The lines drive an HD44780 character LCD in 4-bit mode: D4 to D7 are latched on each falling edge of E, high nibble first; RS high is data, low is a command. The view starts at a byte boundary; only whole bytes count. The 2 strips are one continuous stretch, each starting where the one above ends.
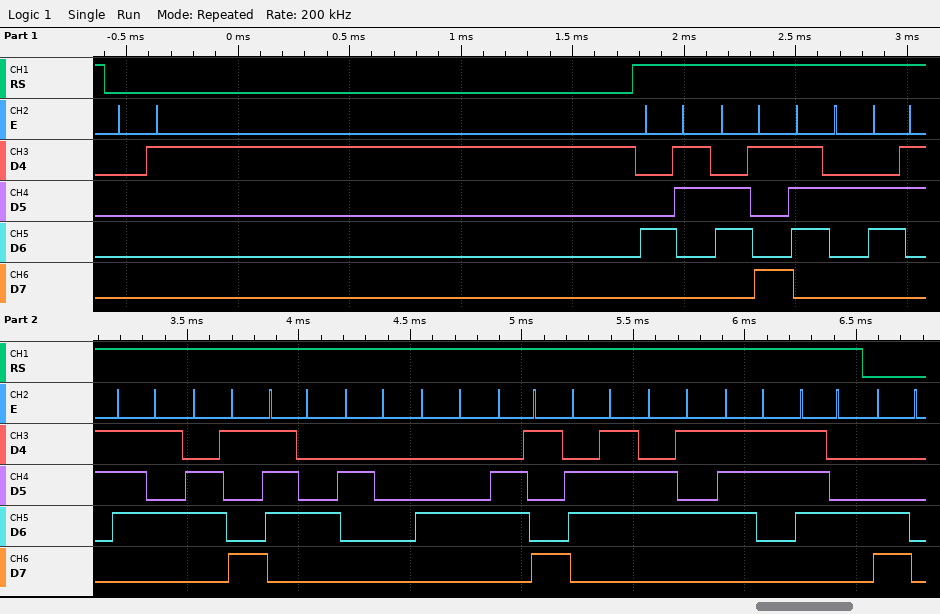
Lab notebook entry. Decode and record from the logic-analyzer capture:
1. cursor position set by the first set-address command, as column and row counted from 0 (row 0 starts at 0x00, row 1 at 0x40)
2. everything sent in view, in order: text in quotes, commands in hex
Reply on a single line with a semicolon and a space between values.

column 0, row 1; 0x01 "Circuit Digest" 0xC0
